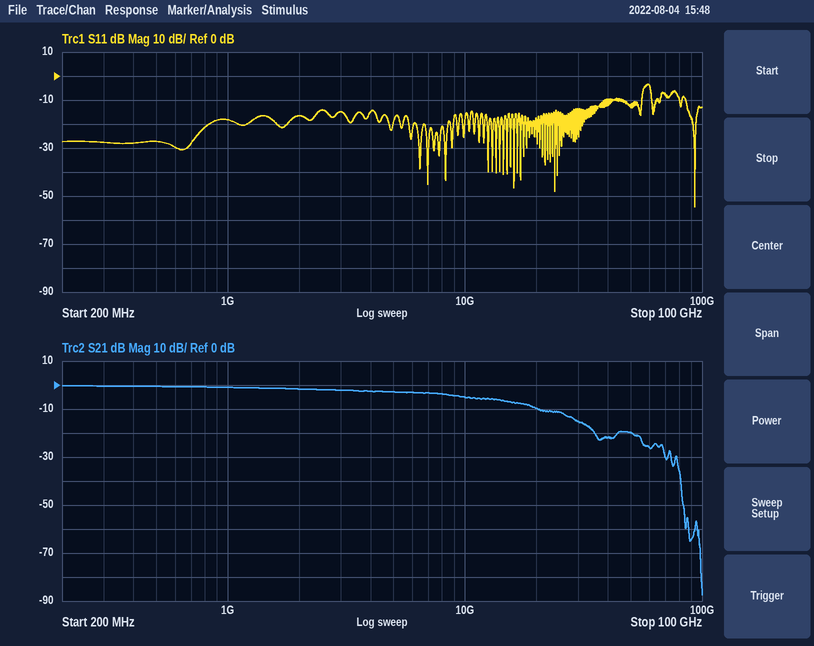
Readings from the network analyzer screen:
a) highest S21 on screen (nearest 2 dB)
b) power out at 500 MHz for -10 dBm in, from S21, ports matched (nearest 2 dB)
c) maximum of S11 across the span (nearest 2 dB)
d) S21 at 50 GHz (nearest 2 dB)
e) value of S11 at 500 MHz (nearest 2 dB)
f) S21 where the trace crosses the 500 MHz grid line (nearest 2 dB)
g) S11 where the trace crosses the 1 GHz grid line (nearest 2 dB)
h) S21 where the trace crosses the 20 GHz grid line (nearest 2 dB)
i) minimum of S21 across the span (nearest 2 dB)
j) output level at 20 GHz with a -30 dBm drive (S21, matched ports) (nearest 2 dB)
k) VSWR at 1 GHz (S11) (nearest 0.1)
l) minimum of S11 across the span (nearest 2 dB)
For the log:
0 dB
-10 dBm
-4 dB
-20 dB
-28 dB
0 dB
-18 dB
-10 dB
-88 dB
-40 dBm
1.3
-54 dB
